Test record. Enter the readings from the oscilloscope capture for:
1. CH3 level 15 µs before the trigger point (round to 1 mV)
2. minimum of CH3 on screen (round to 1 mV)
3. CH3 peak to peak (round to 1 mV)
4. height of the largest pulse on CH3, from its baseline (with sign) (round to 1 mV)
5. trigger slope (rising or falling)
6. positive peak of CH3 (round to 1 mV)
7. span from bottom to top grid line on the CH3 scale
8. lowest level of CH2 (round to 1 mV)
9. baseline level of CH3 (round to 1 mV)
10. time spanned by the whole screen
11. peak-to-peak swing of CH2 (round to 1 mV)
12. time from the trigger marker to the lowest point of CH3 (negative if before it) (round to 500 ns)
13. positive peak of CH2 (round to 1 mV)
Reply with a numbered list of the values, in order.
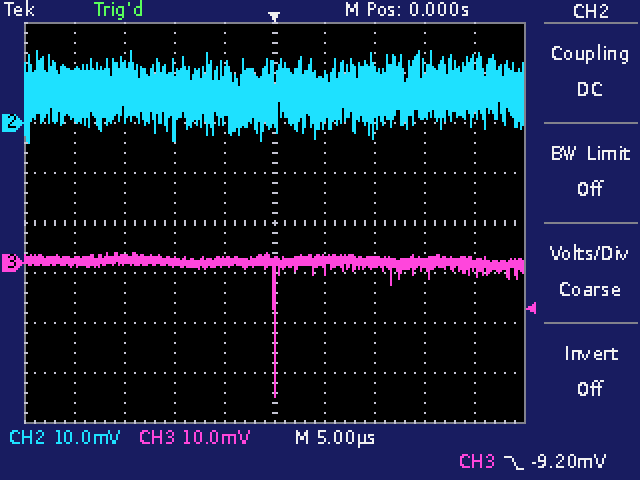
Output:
1. 1 mV
2. -27 mV
3. 29 mV
4. -27 mV
5. falling
6. 2 mV
7. 80 mV
8. -4 mV
9. 0 mV
10. 50 µs
11. 18 mV
12. 0.0 µs
13. 14 mV
